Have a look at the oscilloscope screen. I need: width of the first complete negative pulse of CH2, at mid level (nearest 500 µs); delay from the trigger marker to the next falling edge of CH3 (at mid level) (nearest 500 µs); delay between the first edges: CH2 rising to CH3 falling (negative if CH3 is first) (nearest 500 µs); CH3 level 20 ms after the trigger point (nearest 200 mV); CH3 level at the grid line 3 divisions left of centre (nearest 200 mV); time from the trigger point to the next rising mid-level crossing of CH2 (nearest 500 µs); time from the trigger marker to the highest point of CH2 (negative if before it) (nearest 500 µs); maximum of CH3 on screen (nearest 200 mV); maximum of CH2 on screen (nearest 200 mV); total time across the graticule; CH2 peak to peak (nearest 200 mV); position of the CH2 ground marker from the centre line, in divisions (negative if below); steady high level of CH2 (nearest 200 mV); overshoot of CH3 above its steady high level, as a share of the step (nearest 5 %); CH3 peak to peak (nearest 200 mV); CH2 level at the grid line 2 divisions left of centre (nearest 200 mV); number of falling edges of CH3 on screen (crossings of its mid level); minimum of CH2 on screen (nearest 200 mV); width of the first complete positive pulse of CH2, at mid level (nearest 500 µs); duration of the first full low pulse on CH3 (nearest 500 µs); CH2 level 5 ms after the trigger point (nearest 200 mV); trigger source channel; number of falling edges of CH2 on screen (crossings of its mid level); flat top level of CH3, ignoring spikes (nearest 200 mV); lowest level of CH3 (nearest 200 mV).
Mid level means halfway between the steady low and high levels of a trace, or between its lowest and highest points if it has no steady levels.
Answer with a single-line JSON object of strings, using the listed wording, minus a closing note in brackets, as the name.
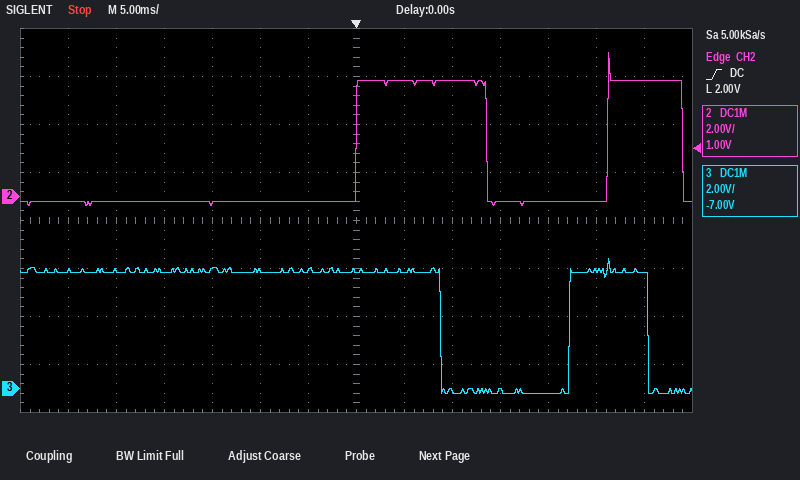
{"width of the first complete negative pulse of CH2, at mid level": "12.5 ms", "delay from the trigger marker to the next falling edge of CH3 (at mid level)": "9.0 ms", "delay between the first edges: CH2 rising to CH3 falling (negative if CH3 is first)": "+9.0 ms", "CH3 level 20 ms after the trigger point": "-200 mV", "CH3 level at the grid line 3 divisions left of centre": "5.0 V", "time from the trigger point to the next rising mid-level crossing of CH2": "26.0 ms", "time from the trigger marker to the highest point of CH2 (negative if before it)": "+26.5 ms", "maximum of CH3 on screen": "5.4 V", "maximum of CH2 on screen": "6.0 V", "total time across the graticule": "70 ms", "CH2 peak to peak": "6.4 V", "position of the CH2 ground marker from the centre line, in divisions": "+0.5 div", "steady high level of CH2": "4.8 V", "overshoot of CH3 above its steady high level, as a share of the step": "10 %", "CH3 peak to peak": "5.6 V", "CH2 level at the grid line 2 divisions left of centre": "-200 mV", "number of falling edges of CH3 on screen": "2", "minimum of CH2 on screen": "-400 mV", "width of the first complete positive pulse of CH2, at mid level": "13.5 ms", "duration of the first full low pulse on CH3": "13.5 ms", "CH2 level 5 ms after the trigger point": "4.8 V", "trigger source channel": "CH2", "number of falling edges of CH2 on screen": "2", "flat top level of CH3, ignoring spikes": "4.8 V", "lowest level of CH3": "-200 mV"}
